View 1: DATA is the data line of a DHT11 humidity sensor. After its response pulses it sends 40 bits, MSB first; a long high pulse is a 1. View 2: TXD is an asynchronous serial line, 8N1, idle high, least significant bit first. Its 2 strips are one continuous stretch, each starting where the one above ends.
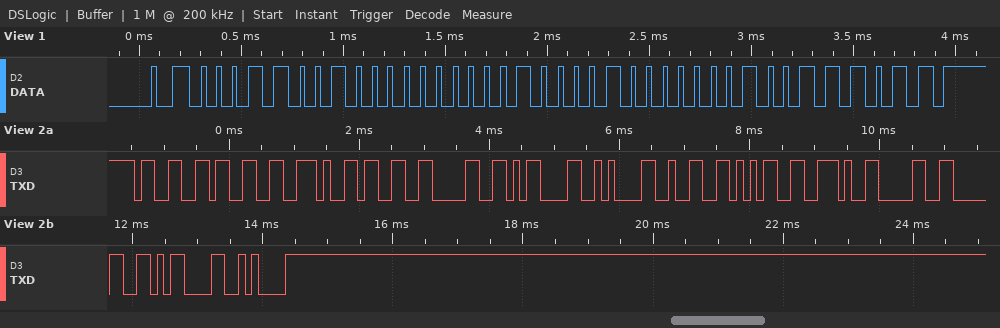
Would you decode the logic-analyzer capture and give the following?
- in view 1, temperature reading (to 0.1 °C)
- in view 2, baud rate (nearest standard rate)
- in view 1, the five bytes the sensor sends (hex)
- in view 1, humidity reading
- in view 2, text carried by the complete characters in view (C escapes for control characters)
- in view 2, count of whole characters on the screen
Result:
33.1 °C
9600 baud
19 00 21 01 3B
25 %
"33.30\r\n25.00\r\n"
14
